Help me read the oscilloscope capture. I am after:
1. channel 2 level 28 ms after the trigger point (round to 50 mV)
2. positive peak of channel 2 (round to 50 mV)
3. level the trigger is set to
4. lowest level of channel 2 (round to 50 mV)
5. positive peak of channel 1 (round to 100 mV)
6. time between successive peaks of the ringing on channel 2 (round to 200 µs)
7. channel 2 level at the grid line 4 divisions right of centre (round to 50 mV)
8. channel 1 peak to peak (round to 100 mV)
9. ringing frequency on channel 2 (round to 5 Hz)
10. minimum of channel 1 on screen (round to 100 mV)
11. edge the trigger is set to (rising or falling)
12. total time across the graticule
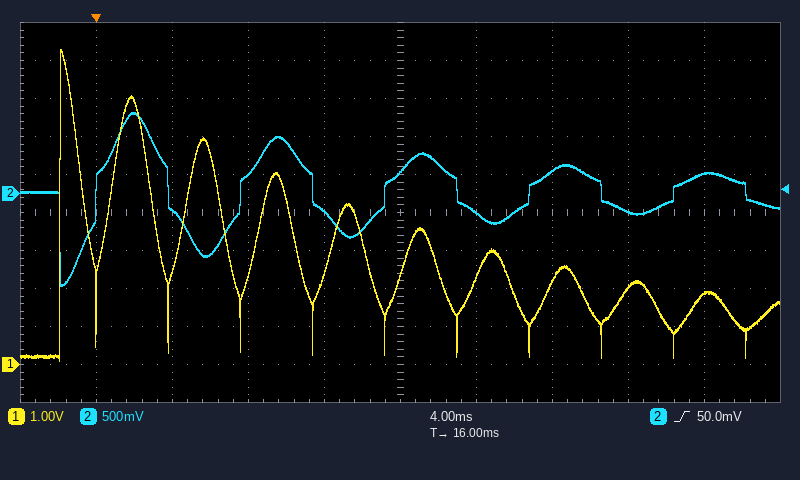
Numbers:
-250 mV
1.05 V
50.0 mV
-1.20 V
8.3 V
7.6 ms
250 mV
8.2 V
130 Hz
100 mV
rising
40 ms
